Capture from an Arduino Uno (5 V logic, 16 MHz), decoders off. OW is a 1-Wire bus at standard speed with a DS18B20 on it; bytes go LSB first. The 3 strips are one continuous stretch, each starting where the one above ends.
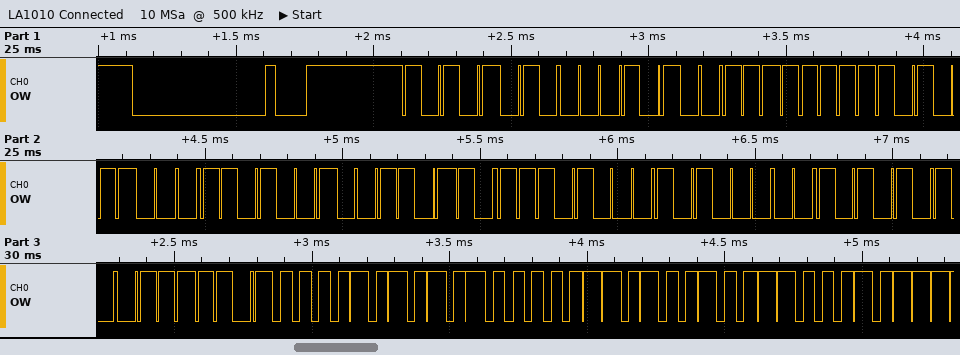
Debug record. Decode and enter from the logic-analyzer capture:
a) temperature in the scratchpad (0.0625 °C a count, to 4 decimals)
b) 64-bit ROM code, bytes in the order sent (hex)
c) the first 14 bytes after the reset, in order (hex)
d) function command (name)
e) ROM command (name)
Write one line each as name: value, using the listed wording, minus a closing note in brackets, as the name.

temperature in the scratchpad: 85.0000 °C
64-bit ROM code, bytes in the order sent: 28 FF 35 96 6C 17 05 55
the first 14 bytes after the reset, in order: 55 28 FF 35 96 6C 17 05 55 BE 50 05 4B 46
function command: Read Scratchpad
ROM command: Match ROM
